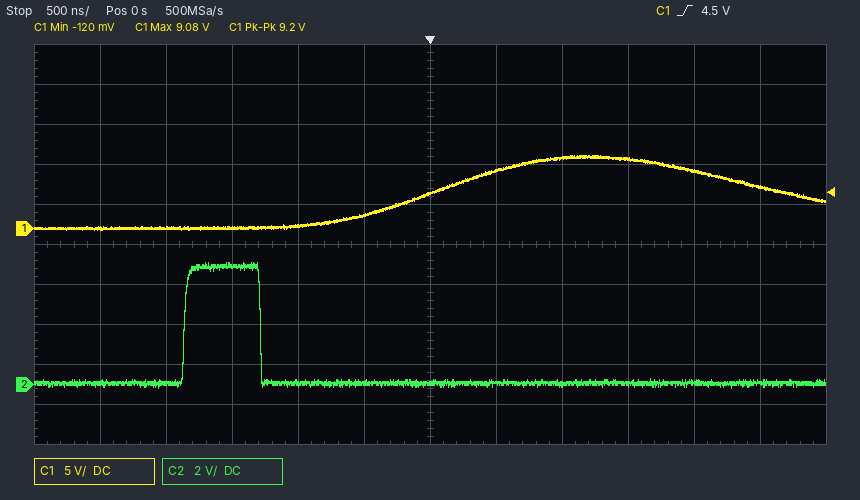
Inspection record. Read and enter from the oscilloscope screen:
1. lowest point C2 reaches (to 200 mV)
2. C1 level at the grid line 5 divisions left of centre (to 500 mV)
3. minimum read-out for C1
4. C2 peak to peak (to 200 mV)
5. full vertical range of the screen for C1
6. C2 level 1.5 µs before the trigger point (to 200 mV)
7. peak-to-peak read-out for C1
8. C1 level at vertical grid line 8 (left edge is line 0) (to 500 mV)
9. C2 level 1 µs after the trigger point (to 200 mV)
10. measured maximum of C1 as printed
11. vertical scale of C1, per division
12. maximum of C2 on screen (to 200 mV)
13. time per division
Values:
-200 mV
0.0 V
-120 mV
6.2 V
50 V
6.0 V
9.2 V
9.0 V
0.0 V
9.08 V
5 V
6.0 V
500 ns
